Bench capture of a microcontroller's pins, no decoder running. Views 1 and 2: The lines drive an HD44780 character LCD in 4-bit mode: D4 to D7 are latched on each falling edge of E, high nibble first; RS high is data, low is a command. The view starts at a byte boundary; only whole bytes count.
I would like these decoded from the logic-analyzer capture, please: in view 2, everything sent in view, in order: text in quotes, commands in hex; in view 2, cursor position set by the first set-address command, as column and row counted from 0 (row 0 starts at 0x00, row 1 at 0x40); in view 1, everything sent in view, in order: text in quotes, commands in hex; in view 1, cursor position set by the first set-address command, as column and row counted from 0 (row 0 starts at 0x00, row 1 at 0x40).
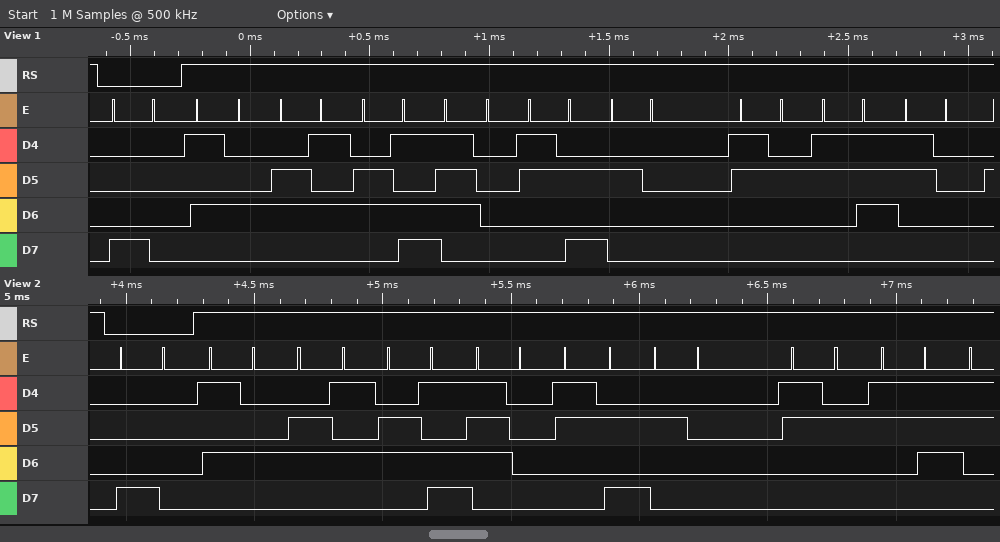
0x80 "Temp: 27"
column 0, row 0
0x80 "Temp: 270"
column 0, row 0
